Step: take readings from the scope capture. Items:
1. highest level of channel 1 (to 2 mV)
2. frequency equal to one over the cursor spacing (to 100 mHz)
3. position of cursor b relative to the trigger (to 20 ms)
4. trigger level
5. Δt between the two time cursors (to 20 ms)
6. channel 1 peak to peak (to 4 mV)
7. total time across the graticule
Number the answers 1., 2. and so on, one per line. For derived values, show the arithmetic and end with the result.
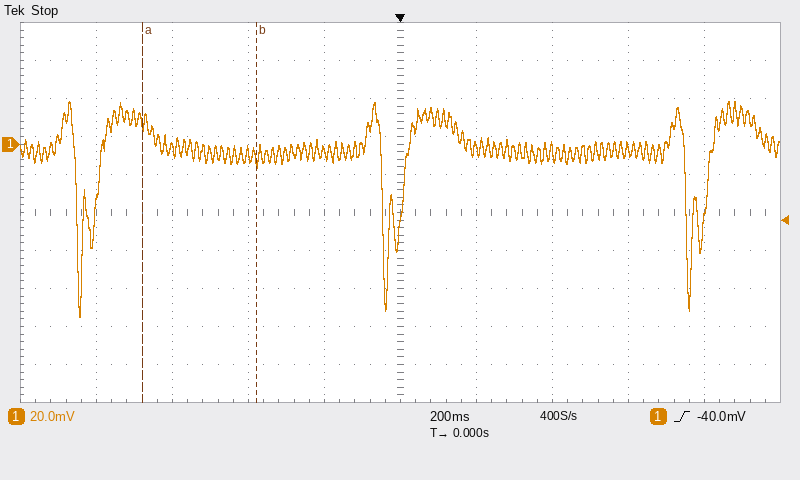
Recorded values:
1. 22 mV
2. 1 / 300 ms ≈ 3.3 Hz
3. -380 ms
4. -40.0 mV
5. 300 ms
6. 112 mV
7. 2 s
